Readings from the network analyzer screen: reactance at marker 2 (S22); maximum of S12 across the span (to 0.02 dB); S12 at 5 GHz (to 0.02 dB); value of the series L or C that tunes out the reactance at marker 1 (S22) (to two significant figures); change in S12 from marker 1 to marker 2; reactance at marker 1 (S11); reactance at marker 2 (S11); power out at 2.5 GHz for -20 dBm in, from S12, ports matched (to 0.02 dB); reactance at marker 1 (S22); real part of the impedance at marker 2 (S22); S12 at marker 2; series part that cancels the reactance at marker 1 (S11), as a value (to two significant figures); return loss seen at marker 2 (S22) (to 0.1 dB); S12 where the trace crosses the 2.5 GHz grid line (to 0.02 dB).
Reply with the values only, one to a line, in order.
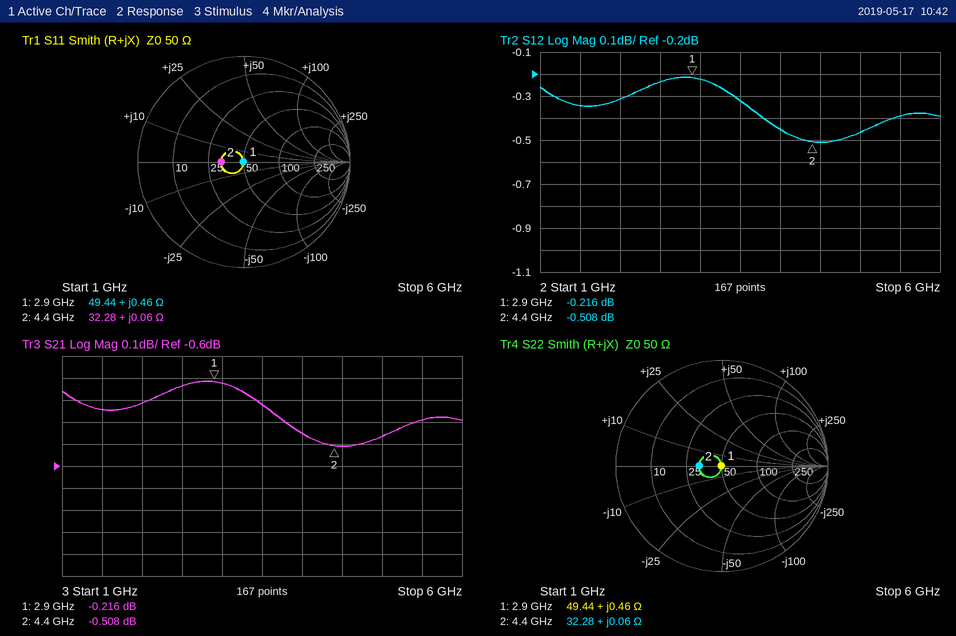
+0.06 Ω
-0.22 dB
-0.46 dB
120 pF
-0.292 dB
+0.46 Ω
+0.06 Ω
-20.24 dBm
+0.46 Ω
32.28 Ω
-0.508 dB
120 pF
13.3 dB
-0.24 dB
